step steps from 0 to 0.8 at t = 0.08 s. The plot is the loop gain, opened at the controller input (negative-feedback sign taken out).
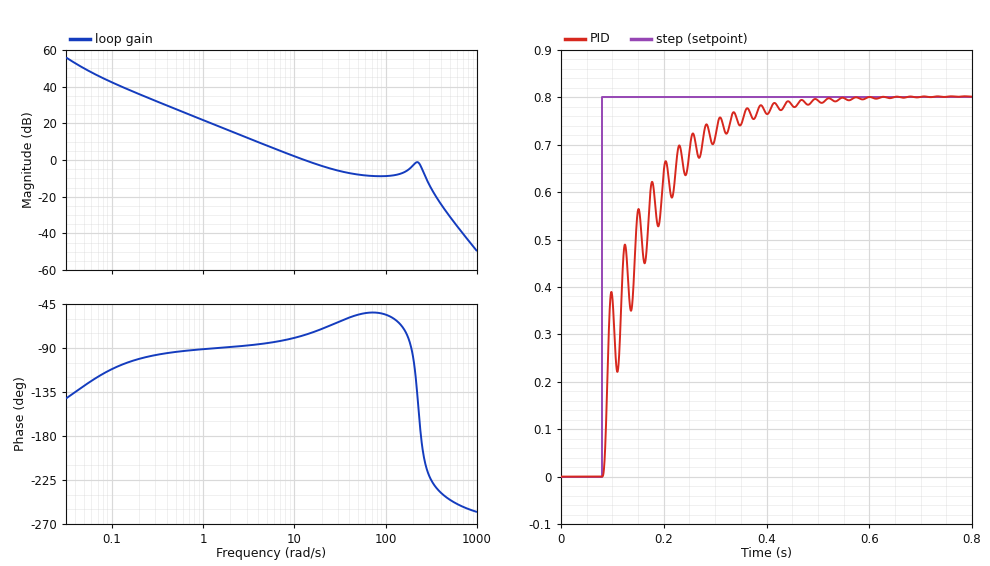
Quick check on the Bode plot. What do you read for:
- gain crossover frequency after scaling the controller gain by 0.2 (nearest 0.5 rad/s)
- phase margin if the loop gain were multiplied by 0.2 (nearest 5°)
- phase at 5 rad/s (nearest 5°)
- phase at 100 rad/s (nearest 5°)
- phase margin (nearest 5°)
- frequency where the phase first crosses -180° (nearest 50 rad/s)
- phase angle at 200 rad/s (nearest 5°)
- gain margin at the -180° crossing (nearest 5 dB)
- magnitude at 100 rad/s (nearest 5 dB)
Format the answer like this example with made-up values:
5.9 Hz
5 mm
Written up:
2.5 rad/s
90°
-85°
-55°
105°
250 rad/s
-100°
5 dB
-10 dB
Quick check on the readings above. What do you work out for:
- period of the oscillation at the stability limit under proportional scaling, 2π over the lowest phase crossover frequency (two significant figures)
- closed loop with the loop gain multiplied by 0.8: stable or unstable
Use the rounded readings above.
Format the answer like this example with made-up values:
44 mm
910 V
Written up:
0.025 s
stable
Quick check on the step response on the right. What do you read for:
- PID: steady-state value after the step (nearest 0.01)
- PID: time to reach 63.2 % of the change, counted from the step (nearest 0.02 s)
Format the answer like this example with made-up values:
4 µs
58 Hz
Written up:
0.80
0.06 s
